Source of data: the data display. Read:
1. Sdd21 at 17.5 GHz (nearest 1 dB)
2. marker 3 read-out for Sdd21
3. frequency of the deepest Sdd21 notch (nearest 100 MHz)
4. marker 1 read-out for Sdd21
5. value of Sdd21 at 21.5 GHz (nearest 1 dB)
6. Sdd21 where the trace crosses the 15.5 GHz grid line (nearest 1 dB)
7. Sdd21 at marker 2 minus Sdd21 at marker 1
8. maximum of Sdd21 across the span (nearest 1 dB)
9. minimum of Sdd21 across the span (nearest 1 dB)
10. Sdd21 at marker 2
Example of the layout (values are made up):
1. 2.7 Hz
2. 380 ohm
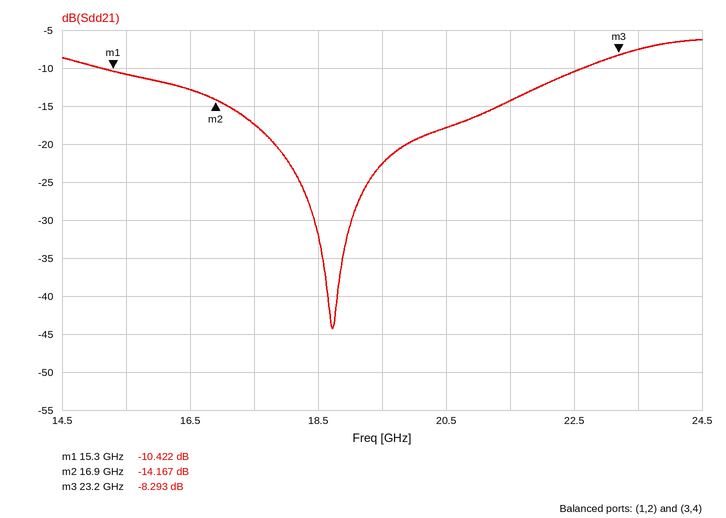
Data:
1. -17 dB
2. -8.293 dB
3. 18.7 GHz
4. -10.422 dB
5. -14 dB
6. -11 dB
7. -3.745 dB
8. -6 dB
9. -44 dB
10. -14.167 dB
